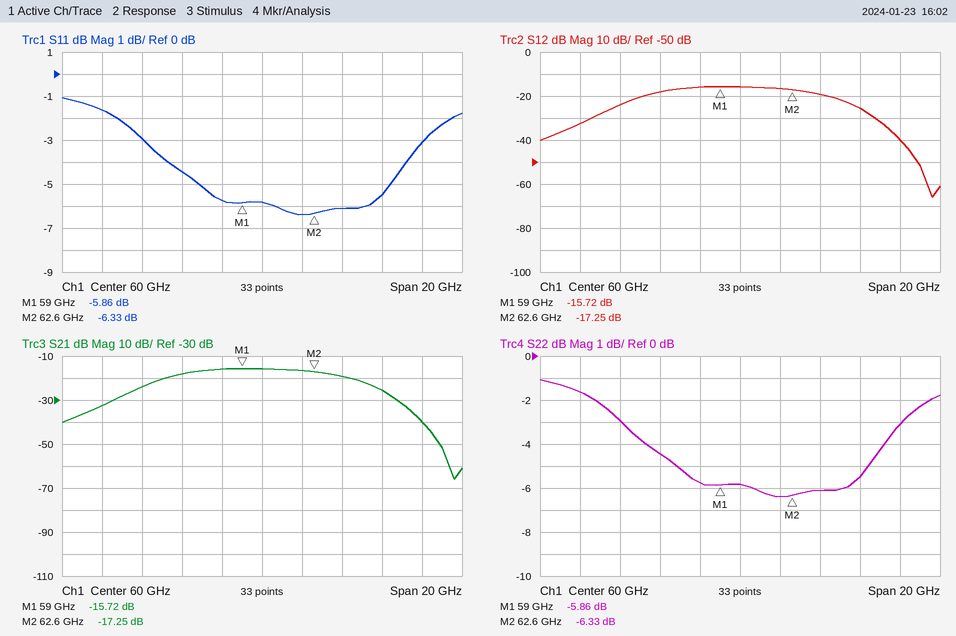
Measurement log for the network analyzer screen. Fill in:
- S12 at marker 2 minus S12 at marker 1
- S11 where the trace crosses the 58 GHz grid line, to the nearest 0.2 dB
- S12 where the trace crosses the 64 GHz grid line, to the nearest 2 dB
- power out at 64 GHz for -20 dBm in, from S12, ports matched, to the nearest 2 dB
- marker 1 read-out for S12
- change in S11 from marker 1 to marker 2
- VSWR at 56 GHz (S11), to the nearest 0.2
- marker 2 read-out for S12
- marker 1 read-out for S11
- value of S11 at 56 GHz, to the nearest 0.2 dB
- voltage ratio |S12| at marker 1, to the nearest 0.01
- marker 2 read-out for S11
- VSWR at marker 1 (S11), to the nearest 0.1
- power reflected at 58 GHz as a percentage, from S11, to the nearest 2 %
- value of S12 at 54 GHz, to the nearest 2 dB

-1.53 dB
-5.8 dB
-20 dB
-40 dBm
-15.72 dB
-0.47 dB
4.0
-17.25 dB
-5.86 dB
-4.4 dB
0.16
-6.33 dB
3.1
26 %
-24 dB
